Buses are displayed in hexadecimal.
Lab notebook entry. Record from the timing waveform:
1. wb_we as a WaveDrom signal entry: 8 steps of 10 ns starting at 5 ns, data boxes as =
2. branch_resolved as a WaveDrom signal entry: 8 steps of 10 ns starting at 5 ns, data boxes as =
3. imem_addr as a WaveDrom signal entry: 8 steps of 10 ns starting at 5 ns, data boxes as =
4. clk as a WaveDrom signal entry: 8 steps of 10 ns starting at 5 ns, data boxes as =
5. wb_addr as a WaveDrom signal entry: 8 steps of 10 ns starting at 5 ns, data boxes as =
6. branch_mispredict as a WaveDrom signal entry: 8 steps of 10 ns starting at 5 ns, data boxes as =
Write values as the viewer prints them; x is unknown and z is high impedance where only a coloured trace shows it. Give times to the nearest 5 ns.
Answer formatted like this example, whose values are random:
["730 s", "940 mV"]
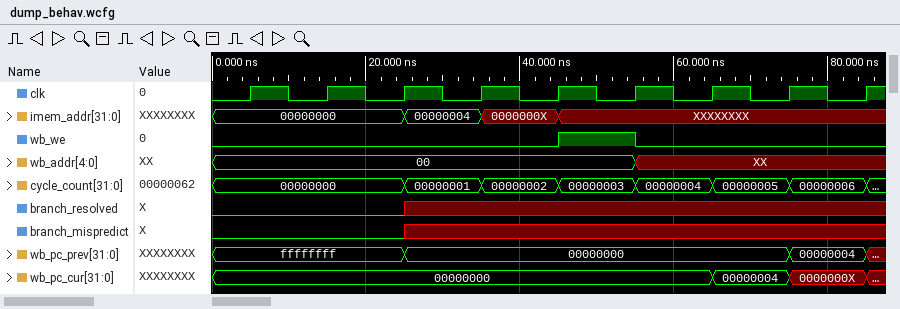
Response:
["{name: 'wb_we', wave: '0...10..'}", "{name: 'branch_resolved', wave: '0.x.....'}", "{name: 'imem_addr', wave: '=.==x...', data: '00000000 00000004 0000000X'}", "{name: 'clk', wave: 'p.......'}", "{name: 'wb_addr', wave: '=....x..', data: '00'}", "{name: 'branch_mispredict', wave: '0.x.....'}"]
